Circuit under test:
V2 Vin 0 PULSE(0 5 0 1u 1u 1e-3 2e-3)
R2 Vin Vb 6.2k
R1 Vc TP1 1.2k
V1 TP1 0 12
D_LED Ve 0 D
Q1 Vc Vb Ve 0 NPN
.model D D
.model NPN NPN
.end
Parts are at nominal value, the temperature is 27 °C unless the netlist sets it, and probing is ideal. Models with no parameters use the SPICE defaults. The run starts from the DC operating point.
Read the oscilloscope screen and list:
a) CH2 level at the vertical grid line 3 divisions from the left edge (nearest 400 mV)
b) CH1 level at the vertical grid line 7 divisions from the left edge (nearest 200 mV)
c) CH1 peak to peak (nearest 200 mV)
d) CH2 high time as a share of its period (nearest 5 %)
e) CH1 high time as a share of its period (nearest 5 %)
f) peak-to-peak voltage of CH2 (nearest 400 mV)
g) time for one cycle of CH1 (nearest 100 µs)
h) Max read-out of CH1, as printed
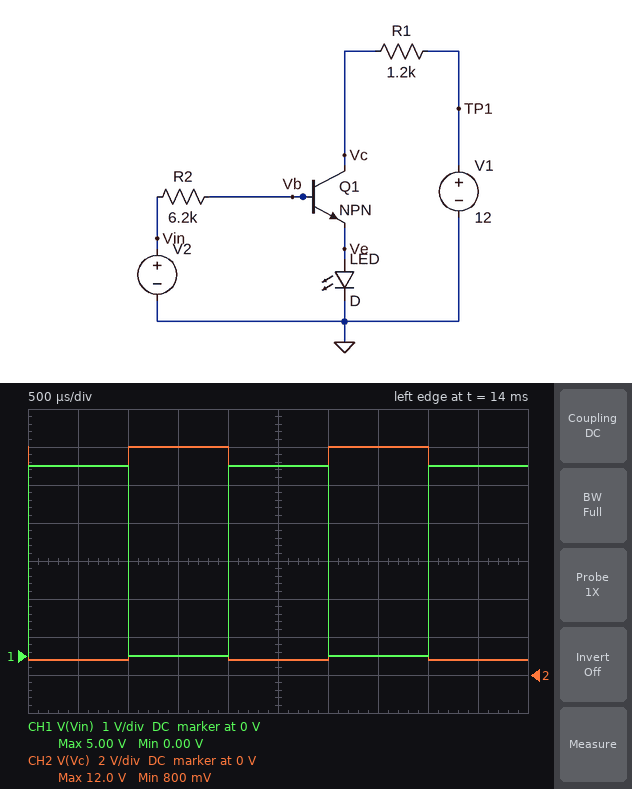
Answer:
12.0 V
0 V
5.0 V
50 %
50 %
11.2 V
2.0 ms
5.00 V
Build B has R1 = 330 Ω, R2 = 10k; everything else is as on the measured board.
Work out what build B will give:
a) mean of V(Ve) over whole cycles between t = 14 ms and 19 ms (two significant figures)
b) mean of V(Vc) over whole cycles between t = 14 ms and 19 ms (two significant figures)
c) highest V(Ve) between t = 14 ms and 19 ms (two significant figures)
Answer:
370 mV
6.5 V
750 mV
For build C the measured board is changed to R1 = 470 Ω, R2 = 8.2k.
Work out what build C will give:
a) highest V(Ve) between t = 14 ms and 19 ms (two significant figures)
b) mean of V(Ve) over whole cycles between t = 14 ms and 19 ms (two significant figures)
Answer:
740 mV
370 mV
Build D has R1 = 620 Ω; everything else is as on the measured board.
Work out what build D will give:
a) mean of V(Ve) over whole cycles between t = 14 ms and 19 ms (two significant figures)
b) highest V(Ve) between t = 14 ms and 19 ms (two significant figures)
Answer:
370 mV
730 mV
